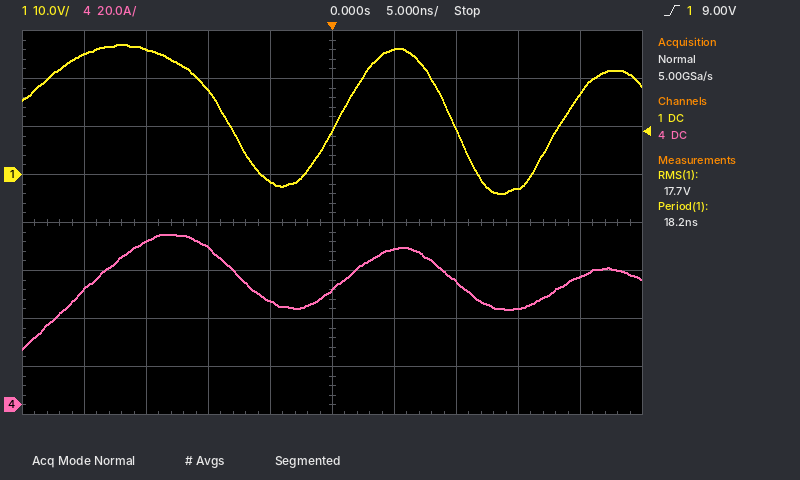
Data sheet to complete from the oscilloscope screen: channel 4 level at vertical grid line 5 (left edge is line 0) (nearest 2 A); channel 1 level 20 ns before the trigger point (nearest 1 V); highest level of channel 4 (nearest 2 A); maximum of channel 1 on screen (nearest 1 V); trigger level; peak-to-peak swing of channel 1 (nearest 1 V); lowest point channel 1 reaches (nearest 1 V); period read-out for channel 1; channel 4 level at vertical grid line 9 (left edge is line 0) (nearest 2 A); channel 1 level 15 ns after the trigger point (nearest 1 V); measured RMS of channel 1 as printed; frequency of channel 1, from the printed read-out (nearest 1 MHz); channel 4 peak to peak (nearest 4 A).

48 A
25 V
72 A
27 V
9.00 V
31 V
-4 V
18.2 ns
54 A
-3 V
17.7 V
55 MHz
48 A
